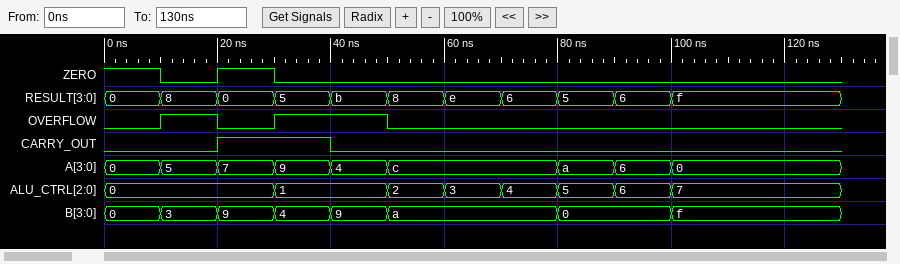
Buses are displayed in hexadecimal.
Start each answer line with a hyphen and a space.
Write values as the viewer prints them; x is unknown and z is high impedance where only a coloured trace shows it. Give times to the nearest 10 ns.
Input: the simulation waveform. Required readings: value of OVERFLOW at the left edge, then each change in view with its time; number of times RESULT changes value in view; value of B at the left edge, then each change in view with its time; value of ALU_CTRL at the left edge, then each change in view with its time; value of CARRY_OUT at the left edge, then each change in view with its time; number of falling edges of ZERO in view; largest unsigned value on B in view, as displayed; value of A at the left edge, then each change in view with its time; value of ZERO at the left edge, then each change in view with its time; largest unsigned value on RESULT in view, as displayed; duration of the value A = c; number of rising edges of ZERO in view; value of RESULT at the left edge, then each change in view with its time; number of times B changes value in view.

- 0, 1 at 10 ns, 0 at 20 ns, 1 at 30 ns, 0 at 50 ns
- 10
- 0, 3 at 10 ns, 9 at 20 ns, 4 at 30 ns, 9 at 40 ns, a at 50 ns, 0 at 80 ns, f at 100 ns
- 0, 1 at 30 ns, 2 at 50 ns, 3 at 60 ns, 4 at 70 ns, 5 at 80 ns, 6 at 90 ns, 7 at 100 ns
- 0, 1 at 20 ns, 0 at 40 ns
- 2
- f
- 0, 5 at 10 ns, 7 at 20 ns, 9 at 30 ns, 4 at 40 ns, c at 50 ns, a at 80 ns, 6 at 90 ns, 0 at 100 ns
- 1, 0 at 10 ns, 1 at 20 ns, 0 at 30 ns
- f
- 30 ns
- 1
- 0, 8 at 10 ns, 0 at 20 ns, 5 at 30 ns, b at 40 ns, 8 at 50 ns, e at 60 ns, 6 at 70 ns, 5 at 80 ns, 6 at 90 ns, f at 100 ns
- 7
